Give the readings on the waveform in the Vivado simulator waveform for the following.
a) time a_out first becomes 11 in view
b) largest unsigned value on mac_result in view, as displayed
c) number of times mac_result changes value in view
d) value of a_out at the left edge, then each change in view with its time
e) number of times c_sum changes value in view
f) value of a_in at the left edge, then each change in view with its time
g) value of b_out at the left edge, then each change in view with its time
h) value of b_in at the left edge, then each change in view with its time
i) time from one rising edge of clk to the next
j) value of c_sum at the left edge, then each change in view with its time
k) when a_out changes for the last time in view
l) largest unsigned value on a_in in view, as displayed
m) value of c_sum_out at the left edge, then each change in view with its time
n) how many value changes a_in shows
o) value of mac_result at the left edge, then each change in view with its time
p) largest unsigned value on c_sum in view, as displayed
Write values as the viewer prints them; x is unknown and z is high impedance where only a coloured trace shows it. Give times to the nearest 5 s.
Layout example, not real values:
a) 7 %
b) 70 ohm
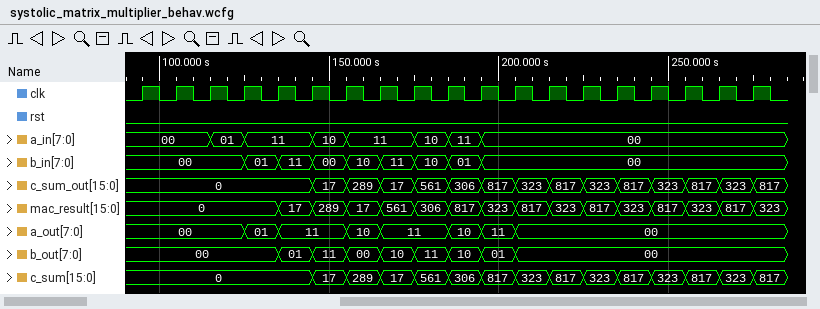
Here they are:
a) 135 s
b) 817
c) 15
d) 00, 01 at 125 s, 11 at 135 s, 10 at 155 s, 11 at 165 s, 10 at 185 s, 11 at 195 s, 00 at 205 s
e) 14
f) 00, 01 at 115 s, 11 at 125 s, 10 at 145 s, 11 at 155 s, 10 at 175 s, 11 at 185 s, 00 at 195 s
g) 00, 01 at 135 s, 11 at 145 s, 00 at 155 s, 10 at 165 s, 11 at 175 s, 10 at 185 s, 01 at 195 s, 00 at 205 s
h) 00, 01 at 125 s, 11 at 135 s, 00 at 145 s, 10 at 155 s, 11 at 165 s, 10 at 175 s, 01 at 185 s, 00 at 195 s
i) 10 s
j) 0, 17 at 145 s, 289 at 155 s, 17 at 165 s, 561 at 175 s, 306 at 185 s, 817 at 195 s, 323 at 205 s, 817 at 215 s, 323 at 225 s, 817 at 235 s, 323 at 245 s, 817 at 255 s, 323 at 265 s, 817 at 275 s
k) 205 s
l) 11
m) 0, 17 at 145 s, 289 at 155 s, 17 at 165 s, 561 at 175 s, 306 at 185 s, 817 at 195 s, 323 at 205 s, 817 at 215 s, 323 at 225 s, 817 at 235 s, 323 at 245 s, 817 at 255 s, 323 at 265 s, 817 at 275 s
n) 7
o) 0, 17 at 135 s, 289 at 145 s, 17 at 155 s, 561 at 165 s, 306 at 175 s, 817 at 185 s, 323 at 195 s, 817 at 205 s, 323 at 215 s, 817 at 225 s, 323 at 235 s, 817 at 245 s, 323 at 255 s, 817 at 265 s, 323 at 275 s
p) 817
